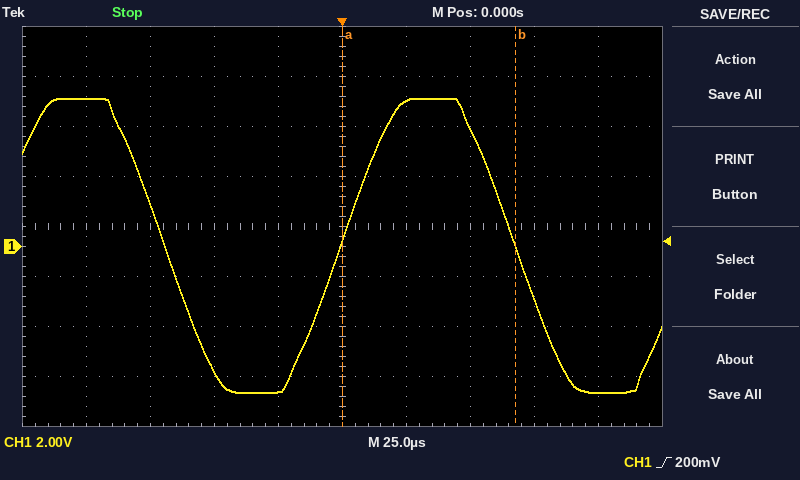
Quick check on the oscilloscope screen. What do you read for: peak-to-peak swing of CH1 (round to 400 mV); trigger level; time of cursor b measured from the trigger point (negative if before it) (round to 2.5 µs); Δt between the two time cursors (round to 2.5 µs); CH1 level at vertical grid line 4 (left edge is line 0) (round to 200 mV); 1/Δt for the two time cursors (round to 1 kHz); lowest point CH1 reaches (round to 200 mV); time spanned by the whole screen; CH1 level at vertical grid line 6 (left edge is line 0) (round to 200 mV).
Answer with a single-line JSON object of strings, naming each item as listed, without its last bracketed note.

{"peak-to-peak swing of CH1": "11.6 V", "trigger level": "200 mV", "time of cursor b measured from the trigger point (negative if before it)": "+67.5 µs", "Δt between the two time cursors": "67.5 µs", "CH1 level at vertical grid line 4 (left edge is line 0)": "-5.8 V", "1/Δt for the two time cursors": "15 kHz", "lowest point CH1 reaches": "-5.8 V", "time spanned by the whole screen": "250 µs", "CH1 level at vertical grid line 6 (left edge is line 0)": "5.8 V"}
